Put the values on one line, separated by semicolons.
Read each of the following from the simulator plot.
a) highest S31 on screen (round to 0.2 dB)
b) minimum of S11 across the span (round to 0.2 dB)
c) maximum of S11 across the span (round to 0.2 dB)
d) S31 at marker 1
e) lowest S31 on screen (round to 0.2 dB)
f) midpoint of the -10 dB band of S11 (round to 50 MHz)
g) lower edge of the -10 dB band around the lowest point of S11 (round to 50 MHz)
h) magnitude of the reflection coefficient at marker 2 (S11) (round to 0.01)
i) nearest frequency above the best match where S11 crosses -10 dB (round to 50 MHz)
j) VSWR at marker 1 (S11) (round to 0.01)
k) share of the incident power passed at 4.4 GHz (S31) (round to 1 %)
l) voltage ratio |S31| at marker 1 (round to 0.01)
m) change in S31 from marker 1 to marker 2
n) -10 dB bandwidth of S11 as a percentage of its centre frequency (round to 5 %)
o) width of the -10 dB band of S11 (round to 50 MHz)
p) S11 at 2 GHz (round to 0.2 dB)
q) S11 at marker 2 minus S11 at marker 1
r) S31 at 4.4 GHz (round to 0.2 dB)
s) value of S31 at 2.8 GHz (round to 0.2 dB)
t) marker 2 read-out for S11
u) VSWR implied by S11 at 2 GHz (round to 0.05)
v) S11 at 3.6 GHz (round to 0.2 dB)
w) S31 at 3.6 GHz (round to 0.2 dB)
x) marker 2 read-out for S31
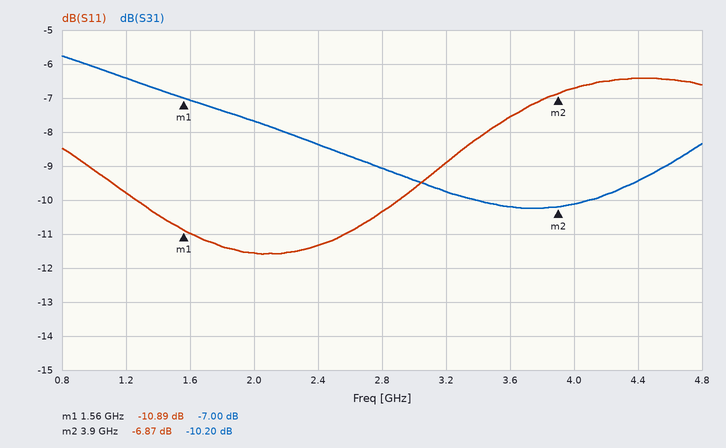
-5.8 dB; -11.6 dB; -6.4 dB; -7.00 dB; -10.2 dB; 2.10 GHz; 1.25 GHz; 0.45; 2.90 GHz; 1.80; 11 %; 0.45; -3.20 dB; 80 %; 1.65 GHz; -11.6 dB; 4.02 dB; -9.4 dB; -9.0 dB; -6.87 dB; 1.70; -7.6 dB; -10.2 dB; -10.20 dB
